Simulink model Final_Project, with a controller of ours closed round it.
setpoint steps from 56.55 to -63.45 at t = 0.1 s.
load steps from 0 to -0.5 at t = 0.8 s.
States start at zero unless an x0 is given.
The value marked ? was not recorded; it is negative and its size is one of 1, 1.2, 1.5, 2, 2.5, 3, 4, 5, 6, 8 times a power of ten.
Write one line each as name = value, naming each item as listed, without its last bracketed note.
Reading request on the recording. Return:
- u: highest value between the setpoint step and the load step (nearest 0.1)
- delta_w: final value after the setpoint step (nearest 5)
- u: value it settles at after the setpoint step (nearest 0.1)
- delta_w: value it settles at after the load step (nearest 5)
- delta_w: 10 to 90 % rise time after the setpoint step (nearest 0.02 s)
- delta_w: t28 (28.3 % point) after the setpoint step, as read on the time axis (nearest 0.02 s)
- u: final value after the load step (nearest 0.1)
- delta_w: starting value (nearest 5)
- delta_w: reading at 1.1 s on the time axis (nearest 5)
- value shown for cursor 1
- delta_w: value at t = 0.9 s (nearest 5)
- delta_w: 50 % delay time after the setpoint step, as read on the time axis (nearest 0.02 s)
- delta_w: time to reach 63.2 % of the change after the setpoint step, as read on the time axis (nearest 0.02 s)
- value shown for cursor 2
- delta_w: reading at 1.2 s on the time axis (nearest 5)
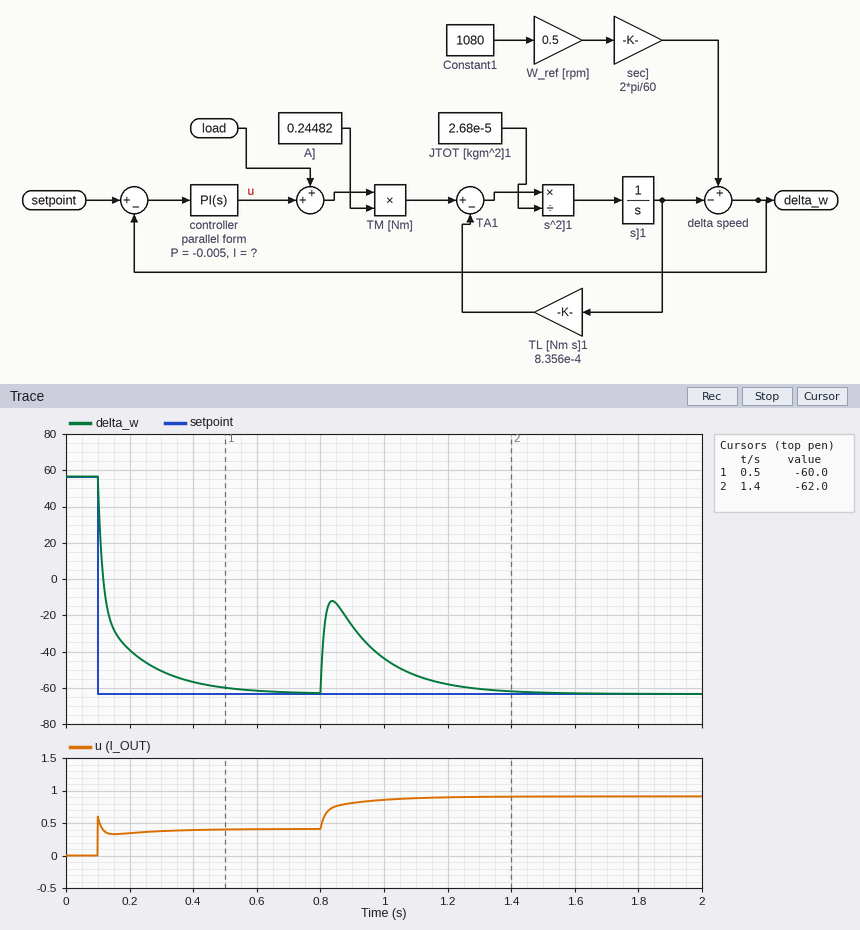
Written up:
u: highest value between the setpoint step and the load step = 0.6
delta_w: final value after the setpoint step = -65
u: value it settles at after the setpoint step = 0.4
delta_w: value it settles at after the load step = -65
delta_w: 10 to 90 % rise time after the setpoint step = 0.20 s
delta_w: t28 (28.3 % point) after the setpoint step, as read on the time axis = 0.10 s
u: final value after the load step = 0.9
delta_w: starting value = 55
delta_w: reading at 1.1 s on the time axis = -55
value shown for cursor 1 = -60.0
delta_w: value at t = 0.9 s = -25
delta_w: 50 % delay time after the setpoint step, as read on the time axis = 0.12 s
delta_w: time to reach 63.2 % of the change after the setpoint step, as read on the time axis = 0.14 s
value shown for cursor 2 = -62.0
delta_w: reading at 1.2 s on the time axis = -60
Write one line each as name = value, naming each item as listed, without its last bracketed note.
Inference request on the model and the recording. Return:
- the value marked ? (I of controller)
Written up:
the value marked ? = -0.05
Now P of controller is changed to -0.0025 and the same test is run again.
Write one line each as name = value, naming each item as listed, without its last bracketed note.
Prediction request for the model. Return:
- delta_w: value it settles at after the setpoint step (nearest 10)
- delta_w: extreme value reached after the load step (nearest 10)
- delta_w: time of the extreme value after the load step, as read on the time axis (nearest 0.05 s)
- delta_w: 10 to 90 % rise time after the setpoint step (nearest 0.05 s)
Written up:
delta_w: value it settles at after the setpoint step = -60
delta_w: extreme value reached after the load step = 0
delta_w: time of the extreme value after the load step, as read on the time axis = 0.85 s
delta_w: 10 to 90 % rise time after the setpoint step = 0.15 s
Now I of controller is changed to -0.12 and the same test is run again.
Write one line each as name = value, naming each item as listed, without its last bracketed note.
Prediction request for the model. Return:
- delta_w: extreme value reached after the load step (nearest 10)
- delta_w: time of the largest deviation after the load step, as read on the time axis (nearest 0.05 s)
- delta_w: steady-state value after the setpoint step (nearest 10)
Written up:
delta_w: extreme value reached after the load step = -20
delta_w: time of the largest deviation after the load step, as read on the time axis = 0.85 s
delta_w: steady-state value after the setpoint step = -60
